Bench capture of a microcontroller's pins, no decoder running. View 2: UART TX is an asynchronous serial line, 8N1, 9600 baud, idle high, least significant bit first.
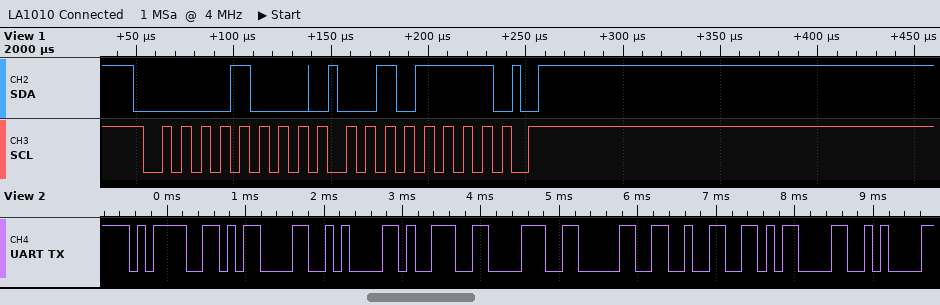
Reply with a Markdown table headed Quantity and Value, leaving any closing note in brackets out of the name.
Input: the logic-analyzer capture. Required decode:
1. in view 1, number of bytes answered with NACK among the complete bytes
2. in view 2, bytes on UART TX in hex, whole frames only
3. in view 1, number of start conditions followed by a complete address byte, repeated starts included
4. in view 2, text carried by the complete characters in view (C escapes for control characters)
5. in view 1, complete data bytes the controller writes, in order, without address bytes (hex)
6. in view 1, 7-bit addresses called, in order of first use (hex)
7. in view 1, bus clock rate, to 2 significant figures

| Quantity | Value |
|---|---|
| in view 1, number of bytes answered with NACK among the complete bytes | 0 |
| in view 2, bytes on UART TX in hex, whole frames only | 3D 0D 0A 39 38 30 32 0D 0A |
| in view 1, number of start conditions followed by a complete address byte, repeated starts included | 1 |
| in view 2, text carried by the complete characters in view | "=\r\n9802\r\n" |
| in view 1, complete data bytes the controller writes, in order, without address bytes | 2F |
| in view 1, 7-bit addresses called, in order of first use | 0x04 |
| in view 1, bus clock rate, to 2 significant figures | 100 kHz |
